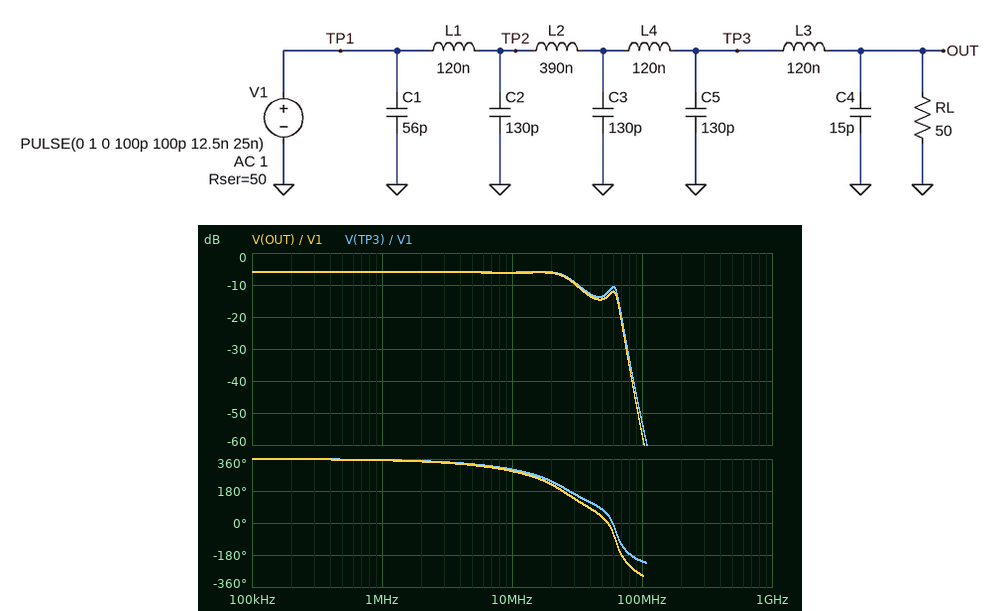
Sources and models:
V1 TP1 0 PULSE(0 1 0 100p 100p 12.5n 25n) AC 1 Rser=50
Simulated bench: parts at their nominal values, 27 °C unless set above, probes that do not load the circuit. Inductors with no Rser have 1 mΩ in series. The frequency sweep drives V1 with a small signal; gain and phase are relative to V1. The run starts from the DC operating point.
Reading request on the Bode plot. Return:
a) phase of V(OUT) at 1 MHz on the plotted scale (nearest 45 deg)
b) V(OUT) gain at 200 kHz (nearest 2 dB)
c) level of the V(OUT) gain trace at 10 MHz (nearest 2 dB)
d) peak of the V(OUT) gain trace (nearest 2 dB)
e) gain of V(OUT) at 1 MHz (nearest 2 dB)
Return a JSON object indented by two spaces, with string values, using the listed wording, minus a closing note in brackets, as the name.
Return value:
{
  "phase of V(OUT) at 1 MHz on the plotted scale": "360 deg",
  "V(OUT) gain at 200 kHz": "-6 dB",
  "level of the V(OUT) gain trace at 10 MHz": "-6 dB",
  "peak of the V(OUT) gain trace": "-6 dB",
  "gain of V(OUT) at 1 MHz": "-6 dB"
}
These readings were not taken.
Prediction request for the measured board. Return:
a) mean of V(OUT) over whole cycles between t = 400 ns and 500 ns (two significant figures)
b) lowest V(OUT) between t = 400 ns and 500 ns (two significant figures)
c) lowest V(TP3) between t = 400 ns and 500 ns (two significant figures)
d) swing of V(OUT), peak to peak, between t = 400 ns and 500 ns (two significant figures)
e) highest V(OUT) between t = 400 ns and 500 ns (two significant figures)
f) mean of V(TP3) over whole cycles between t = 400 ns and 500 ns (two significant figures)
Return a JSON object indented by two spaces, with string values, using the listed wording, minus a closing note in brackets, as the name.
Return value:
{
  "mean of V(OUT) over whole cycles between t = 400 ns and 500 ns": "250 mV",
  "lowest V(OUT) between t = 400 ns and 500 ns": "120 mV",
  "lowest V(TP3) between t = 400 ns and 500 ns": "110 mV",
  "swing of V(OUT), peak to peak, between t = 400 ns and 500 ns": "270 mV",
  "highest V(OUT) between t = 400 ns and 500 ns": "390 mV",
  "mean of V(TP3) over whole cycles between t = 400 ns and 500 ns": "250 mV"
}
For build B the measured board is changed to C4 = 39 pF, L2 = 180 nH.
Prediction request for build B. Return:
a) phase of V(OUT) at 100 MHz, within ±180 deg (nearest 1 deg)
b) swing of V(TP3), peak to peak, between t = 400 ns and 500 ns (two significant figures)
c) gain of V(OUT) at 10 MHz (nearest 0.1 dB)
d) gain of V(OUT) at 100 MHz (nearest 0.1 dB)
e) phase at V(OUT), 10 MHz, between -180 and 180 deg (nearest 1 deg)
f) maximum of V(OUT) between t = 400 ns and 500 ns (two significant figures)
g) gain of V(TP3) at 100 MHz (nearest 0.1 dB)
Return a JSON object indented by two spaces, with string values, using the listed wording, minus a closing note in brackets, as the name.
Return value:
{
  "phase of V(OUT) at 100 MHz, within ±180 deg": "25 deg",
  "swing of V(TP3), peak to peak, between t = 400 ns and 500 ns": "510 mV",
  "gain of V(OUT) at 10 MHz": "-6.5 dB",
  "gain of V(OUT) at 100 MHz": "-48.3 dB",
  "phase at V(OUT), 10 MHz, between -180 and 180 deg": "-60 deg",
  "maximum of V(OUT) between t = 400 ns and 500 ns": "530 mV",
  "gain of V(TP3) at 100 MHz": "-43.5 dB"
}
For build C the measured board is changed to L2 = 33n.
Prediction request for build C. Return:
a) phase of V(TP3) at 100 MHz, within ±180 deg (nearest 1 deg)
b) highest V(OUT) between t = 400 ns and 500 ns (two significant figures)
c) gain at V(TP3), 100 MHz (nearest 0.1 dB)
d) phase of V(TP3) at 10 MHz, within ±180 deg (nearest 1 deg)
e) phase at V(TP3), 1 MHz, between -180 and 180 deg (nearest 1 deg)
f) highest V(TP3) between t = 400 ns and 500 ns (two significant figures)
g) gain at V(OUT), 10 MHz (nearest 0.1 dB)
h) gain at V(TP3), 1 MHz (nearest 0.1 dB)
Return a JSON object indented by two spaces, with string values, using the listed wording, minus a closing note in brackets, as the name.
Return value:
{
  "phase of V(TP3) at 100 MHz, within ±180 deg": "-41 deg",
  "highest V(OUT) between t = 400 ns and 500 ns": "540 mV",
  "gain at V(TP3), 100 MHz": "-26.3 dB",
  "phase of V(TP3) at 10 MHz, within ±180 deg": "-44 deg",
  "phase at V(TP3), 1 MHz, between -180 and 180 deg": "-5 deg",
  "highest V(TP3) between t = 400 ns and 500 ns": "570 mV",
  "gain at V(OUT), 10 MHz": "-6.8 dB",
  "gain at V(TP3), 1 MHz": "-6.0 dB"
}
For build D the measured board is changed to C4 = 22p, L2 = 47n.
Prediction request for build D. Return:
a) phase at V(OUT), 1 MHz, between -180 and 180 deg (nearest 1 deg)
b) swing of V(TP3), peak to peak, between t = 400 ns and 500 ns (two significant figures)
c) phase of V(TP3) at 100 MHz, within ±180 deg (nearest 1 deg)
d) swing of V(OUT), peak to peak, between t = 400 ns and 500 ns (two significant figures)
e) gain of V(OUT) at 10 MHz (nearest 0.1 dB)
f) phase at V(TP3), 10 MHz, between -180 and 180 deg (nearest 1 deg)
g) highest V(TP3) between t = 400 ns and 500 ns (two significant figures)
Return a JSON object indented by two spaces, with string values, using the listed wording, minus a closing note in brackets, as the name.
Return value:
{
  "phase at V(OUT), 1 MHz, between -180 and 180 deg": "-6 deg",
  "swing of V(TP3), peak to peak, between t = 400 ns and 500 ns": "620 mV",
  "phase of V(TP3) at 100 MHz, within ±180 deg": "-74 deg",
  "swing of V(OUT), peak to peak, between t = 400 ns and 500 ns": "600 mV",
  "gain of V(OUT) at 10 MHz": "-6.8 dB",
  "phase at V(TP3), 10 MHz, between -180 and 180 deg": "-45 deg",
  "highest V(TP3) between t = 400 ns and 500 ns": "560 mV"
}
